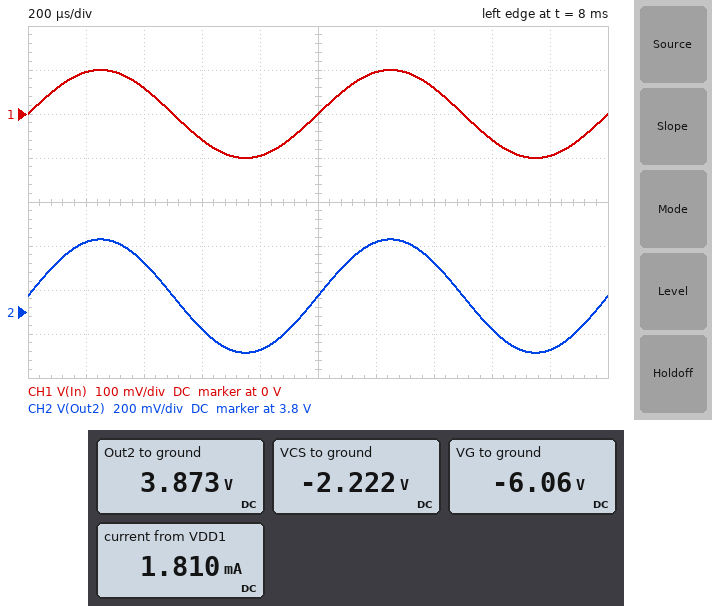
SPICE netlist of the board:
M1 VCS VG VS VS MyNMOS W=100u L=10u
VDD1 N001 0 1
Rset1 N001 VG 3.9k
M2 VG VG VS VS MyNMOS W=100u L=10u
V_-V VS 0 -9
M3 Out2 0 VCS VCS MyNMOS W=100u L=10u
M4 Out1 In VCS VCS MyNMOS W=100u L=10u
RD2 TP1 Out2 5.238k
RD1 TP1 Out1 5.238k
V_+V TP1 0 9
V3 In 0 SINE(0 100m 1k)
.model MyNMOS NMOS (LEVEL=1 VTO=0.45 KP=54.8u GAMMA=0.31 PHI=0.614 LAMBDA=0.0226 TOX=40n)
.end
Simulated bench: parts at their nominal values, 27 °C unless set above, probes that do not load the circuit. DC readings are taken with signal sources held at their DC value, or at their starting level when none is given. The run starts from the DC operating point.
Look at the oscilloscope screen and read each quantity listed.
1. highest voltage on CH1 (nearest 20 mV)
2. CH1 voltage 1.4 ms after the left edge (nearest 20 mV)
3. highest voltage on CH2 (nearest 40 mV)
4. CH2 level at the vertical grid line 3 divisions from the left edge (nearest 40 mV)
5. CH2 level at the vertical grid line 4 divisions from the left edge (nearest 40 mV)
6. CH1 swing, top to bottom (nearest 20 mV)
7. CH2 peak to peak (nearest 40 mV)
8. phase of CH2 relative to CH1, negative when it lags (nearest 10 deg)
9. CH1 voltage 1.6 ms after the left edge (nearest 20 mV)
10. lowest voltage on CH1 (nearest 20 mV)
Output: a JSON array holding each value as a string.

["100 mV", "60 mV", "4.12 V", "3.72 V", "3.64 V", "200 mV", "520 mV", "0 deg", "-60 mV", "-100 mV"]
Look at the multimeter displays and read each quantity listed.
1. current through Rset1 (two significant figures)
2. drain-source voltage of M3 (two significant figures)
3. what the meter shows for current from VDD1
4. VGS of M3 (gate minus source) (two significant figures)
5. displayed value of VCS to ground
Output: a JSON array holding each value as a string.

["1.8 mA", "6.1 V", "1.810 mA", "2.2 V", "-2.222 V"]
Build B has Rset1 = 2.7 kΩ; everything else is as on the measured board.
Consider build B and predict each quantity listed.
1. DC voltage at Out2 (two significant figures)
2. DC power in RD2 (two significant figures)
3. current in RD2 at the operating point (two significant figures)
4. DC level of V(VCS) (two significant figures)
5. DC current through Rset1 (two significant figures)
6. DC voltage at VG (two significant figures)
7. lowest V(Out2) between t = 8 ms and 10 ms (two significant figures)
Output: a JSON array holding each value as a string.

["2.1 V", "9.0 mW", "1.3 mA", "-2.5 V", "2.5 mA", "-5.7 V", "1.8 V"]
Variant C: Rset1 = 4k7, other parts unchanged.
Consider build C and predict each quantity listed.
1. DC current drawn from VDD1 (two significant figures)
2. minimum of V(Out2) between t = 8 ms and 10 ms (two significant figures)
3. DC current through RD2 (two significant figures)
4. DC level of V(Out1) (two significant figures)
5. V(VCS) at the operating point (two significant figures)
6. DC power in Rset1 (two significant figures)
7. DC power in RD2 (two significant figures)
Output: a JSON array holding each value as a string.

["1.5 mA", "4.4 V", "840 µA", "4.6 V", "-2.1 V", "11 mW", "3.7 mW"]
